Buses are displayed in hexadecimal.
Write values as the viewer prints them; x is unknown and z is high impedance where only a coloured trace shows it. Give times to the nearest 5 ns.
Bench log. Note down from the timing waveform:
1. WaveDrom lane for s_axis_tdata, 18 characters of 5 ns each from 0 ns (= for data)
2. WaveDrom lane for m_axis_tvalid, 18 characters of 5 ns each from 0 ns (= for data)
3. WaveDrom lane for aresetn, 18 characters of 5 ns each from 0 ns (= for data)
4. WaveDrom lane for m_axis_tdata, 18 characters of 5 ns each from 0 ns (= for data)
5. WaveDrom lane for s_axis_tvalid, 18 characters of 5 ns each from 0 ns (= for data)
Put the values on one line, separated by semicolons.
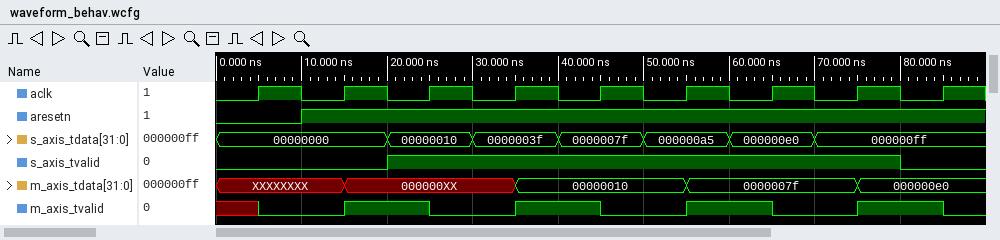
{name: 's_axis_tdata', wave: '=...=.=.=.=.=.=...', data: '00000000 00000010 0000003f 0000007f 000000a5 000000e0 000000ff'}; {name: 'm_axis_tvalid', wave: 'x0.1.0.1.0.1.0.1.0'}; {name: 'aresetn', wave: '0.1...............'}; {name: 'm_axis_tdata', wave: 'x..=...=...=...=..', data: '000000XX 00000010 0000007f 000000e0'}; {name: 's_axis_tvalid', wave: '0...1...........0.'}
